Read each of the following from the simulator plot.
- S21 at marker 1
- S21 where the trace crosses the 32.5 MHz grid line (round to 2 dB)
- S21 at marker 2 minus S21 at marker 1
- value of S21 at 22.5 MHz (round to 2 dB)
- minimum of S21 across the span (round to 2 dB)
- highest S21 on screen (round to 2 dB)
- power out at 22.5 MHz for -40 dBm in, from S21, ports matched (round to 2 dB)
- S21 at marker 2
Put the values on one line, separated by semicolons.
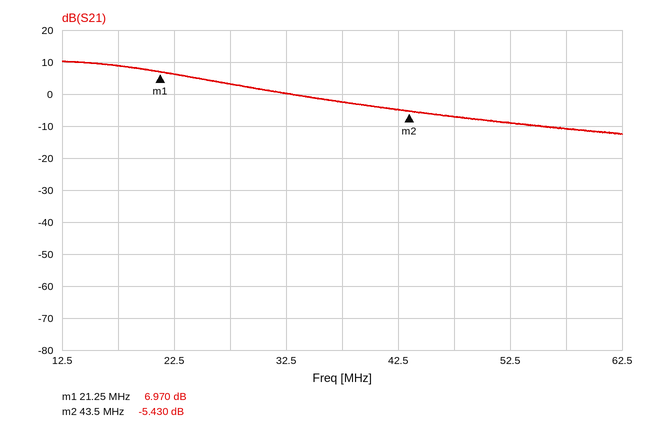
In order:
6.970 dB; 0 dB; -12.400 dB; 6 dB; -12 dB; 10 dB; -34 dBm; -5.430 dB
